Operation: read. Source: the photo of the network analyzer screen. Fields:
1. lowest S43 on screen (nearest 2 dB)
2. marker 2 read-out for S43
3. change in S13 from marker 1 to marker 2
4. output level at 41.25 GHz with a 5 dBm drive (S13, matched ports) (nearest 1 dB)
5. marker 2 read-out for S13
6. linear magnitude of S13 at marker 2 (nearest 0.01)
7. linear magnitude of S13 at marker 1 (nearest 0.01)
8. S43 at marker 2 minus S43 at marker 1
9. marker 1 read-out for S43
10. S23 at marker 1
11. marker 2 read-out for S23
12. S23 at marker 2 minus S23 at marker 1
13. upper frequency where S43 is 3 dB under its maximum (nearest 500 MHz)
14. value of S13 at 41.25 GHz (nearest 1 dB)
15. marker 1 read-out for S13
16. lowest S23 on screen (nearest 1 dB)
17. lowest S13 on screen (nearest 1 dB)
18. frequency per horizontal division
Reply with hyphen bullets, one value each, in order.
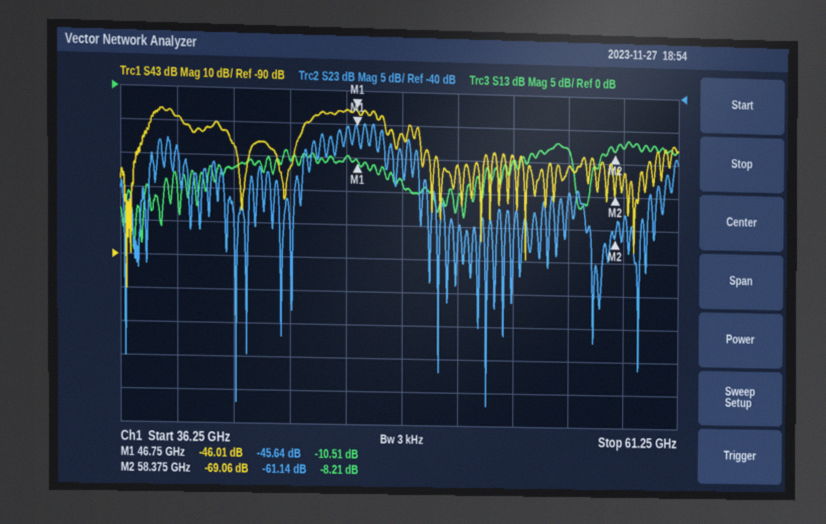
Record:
- -100 dB
- -69.06 dB
- 2.30 dB
- -7 dBm
- -8.21 dB
- 0.39
- 0.30
- -23.05 dB
- -46.01 dB
- -45.64 dB
- -61.14 dB
- -15.50 dB
- 48.0 GHz
- -12 dB
- -10.51 dB
- -87 dB
- -24 dB
- 2.5 GHz
